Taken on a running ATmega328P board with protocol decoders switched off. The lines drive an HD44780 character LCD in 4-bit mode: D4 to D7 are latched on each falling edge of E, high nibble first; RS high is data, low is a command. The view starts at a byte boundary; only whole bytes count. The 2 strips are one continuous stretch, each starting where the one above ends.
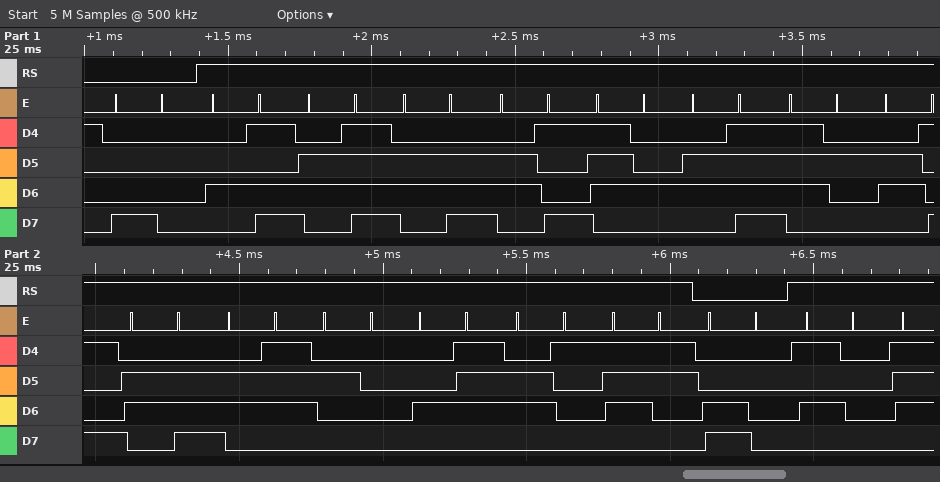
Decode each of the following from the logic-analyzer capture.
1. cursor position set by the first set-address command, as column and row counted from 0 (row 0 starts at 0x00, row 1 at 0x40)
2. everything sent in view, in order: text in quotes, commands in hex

column 0, row 0
0x80 "Monitoring Gas" 0xC0 "P"
